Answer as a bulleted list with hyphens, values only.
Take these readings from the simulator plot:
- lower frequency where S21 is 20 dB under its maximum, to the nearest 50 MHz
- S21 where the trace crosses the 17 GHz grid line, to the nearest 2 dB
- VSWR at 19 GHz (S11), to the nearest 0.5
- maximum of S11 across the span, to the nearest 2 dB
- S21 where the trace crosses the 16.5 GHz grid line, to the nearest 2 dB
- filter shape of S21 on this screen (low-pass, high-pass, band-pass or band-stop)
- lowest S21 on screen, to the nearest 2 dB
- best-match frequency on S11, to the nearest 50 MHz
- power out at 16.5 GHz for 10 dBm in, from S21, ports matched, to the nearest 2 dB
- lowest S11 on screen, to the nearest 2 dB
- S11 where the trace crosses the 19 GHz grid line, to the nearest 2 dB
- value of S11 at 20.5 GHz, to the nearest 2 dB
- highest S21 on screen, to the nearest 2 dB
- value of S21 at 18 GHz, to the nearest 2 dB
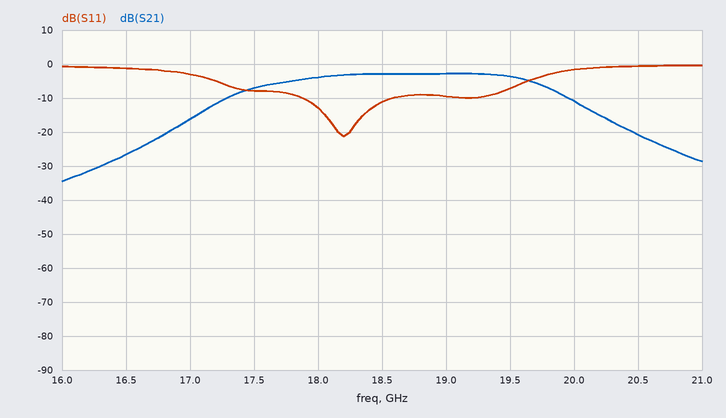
- 16.70 GHz
- -16 dB
- 2.0
- 0 dB
- -26 dB
- band-pass
- -34 dB
- 18.20 GHz
- -16 dBm
- -22 dB
- -10 dB
- 0 dB
- -2 dB
- -4 dB
